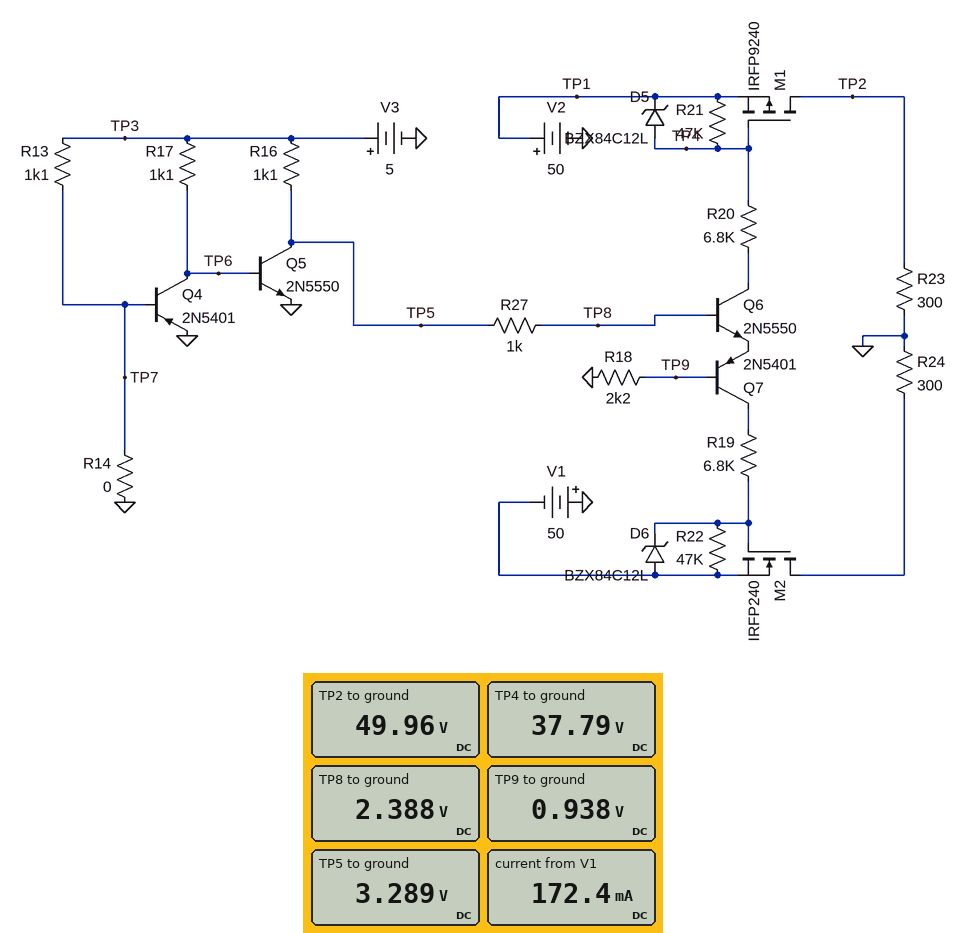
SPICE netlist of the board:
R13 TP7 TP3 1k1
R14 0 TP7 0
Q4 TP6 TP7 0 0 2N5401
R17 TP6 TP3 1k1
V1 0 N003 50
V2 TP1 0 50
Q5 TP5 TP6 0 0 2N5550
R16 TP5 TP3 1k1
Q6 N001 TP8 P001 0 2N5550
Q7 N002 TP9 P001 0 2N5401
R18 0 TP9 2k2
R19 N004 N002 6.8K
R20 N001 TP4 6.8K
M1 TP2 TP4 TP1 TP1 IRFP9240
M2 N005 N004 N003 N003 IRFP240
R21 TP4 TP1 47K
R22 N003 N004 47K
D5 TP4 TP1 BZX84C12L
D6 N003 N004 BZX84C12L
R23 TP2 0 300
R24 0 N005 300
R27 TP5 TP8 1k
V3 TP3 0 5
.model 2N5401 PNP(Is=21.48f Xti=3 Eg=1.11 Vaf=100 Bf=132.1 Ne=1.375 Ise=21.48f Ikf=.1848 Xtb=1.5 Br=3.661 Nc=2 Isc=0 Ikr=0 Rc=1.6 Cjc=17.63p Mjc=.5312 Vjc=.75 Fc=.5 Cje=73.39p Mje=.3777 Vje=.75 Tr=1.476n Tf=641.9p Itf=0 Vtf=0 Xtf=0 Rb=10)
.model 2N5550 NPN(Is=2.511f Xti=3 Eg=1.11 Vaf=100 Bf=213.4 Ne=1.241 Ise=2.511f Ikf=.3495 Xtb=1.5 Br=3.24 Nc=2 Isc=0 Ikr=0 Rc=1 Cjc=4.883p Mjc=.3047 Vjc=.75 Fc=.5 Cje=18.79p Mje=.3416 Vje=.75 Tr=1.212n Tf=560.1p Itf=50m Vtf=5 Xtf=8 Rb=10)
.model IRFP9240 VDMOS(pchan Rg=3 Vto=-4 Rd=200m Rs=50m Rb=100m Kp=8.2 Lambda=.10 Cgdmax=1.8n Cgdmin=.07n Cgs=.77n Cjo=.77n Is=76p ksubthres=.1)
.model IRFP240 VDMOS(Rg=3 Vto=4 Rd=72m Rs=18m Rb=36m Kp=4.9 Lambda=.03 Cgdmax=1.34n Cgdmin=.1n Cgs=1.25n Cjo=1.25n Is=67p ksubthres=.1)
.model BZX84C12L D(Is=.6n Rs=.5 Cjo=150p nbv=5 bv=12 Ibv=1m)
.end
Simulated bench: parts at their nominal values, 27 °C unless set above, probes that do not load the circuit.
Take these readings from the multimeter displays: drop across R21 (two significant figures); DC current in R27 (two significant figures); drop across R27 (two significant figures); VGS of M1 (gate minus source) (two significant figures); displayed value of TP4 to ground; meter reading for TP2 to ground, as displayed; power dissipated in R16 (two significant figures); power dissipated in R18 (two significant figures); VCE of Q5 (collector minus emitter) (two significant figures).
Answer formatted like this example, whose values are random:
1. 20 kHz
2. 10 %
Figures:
1. 12 V
2. 900 µA
3. 900 mV
4. -12 V
5. 37.79 V
6. 49.96 V
7. 2.7 mW
8. 400 µW
9. 3.3 V
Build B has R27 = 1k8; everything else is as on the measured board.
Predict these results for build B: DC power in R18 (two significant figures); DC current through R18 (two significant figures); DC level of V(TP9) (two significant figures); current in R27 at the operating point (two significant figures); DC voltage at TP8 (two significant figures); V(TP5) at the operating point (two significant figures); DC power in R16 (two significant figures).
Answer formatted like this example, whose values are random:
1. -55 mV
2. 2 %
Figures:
1. 230 µW
2. 320 µA
3. 710 mV
4. 730 µA
5. 2.2 V
6. 3.5 V
7. 2.1 mW
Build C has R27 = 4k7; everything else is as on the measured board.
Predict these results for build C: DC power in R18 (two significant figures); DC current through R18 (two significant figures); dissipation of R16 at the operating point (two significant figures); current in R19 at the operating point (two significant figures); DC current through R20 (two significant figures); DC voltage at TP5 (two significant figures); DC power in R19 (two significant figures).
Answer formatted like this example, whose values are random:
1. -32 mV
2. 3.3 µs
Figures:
1. 47 µW
2. 150 µA
3. 1.3 mW
4. 5.7 mA
5. 5.4 mA
6. 3.8 V
7. 220 mW
